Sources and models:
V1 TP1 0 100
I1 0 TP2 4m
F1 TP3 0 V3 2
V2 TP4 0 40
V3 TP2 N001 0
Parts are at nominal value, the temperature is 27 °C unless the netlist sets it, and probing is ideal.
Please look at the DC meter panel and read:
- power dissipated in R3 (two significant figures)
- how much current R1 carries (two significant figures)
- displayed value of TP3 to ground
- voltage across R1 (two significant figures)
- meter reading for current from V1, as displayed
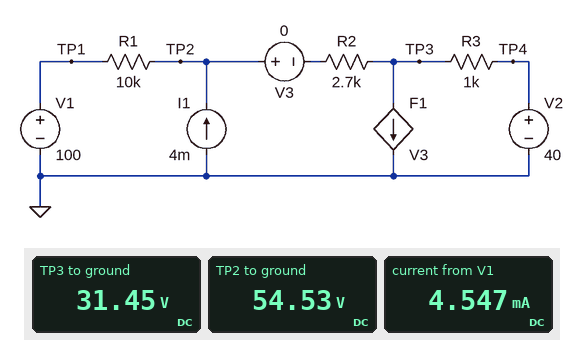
73 mW
4.5 mA
31.45 V
45 V
4.547 mA
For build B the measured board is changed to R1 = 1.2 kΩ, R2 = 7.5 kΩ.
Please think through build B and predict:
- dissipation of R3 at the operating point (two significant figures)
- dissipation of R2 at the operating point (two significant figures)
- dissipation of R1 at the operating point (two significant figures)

71 mW
530 mW
23 mW
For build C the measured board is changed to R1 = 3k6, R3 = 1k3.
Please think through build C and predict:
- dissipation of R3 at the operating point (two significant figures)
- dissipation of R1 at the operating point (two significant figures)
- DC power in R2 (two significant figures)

290 mW
430 mW
600 mW
